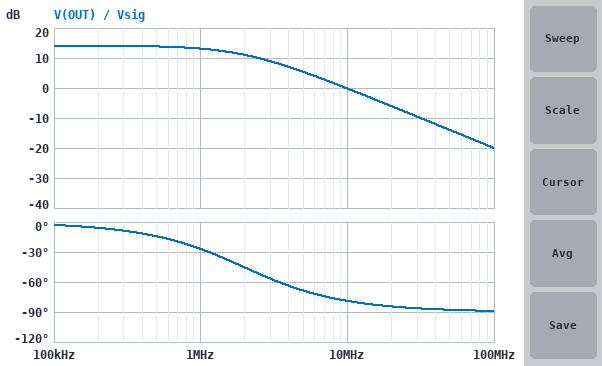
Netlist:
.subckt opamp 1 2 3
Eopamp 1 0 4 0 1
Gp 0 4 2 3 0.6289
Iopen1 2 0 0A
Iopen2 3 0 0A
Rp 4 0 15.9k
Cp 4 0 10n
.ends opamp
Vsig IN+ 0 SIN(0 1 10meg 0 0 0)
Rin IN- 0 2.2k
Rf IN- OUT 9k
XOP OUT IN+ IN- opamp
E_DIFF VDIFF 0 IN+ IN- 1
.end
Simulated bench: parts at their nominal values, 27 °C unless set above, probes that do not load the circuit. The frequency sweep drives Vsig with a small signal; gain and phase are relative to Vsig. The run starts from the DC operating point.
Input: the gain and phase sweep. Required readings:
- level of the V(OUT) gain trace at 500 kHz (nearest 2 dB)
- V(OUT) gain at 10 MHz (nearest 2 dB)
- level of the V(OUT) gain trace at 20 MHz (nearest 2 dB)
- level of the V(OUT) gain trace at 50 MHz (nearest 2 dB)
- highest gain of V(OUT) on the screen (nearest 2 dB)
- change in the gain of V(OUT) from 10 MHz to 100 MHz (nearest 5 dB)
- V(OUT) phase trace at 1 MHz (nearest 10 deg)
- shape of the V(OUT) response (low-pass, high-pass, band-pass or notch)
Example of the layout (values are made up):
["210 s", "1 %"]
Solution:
["14 dB", "0 dB", "-6 dB", "-14 dB", "14 dB", "-20 dB", "-30 deg", "low-pass"]
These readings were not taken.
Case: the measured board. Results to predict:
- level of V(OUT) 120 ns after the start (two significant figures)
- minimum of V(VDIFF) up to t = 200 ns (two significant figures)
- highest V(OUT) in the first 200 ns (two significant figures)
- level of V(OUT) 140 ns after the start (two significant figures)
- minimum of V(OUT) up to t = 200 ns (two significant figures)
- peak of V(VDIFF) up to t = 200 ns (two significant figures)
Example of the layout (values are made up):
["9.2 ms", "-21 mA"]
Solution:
["100 mV", "-1.1 V", "1.5 V", "1.1 V", "-900 mV", "940 mV"]
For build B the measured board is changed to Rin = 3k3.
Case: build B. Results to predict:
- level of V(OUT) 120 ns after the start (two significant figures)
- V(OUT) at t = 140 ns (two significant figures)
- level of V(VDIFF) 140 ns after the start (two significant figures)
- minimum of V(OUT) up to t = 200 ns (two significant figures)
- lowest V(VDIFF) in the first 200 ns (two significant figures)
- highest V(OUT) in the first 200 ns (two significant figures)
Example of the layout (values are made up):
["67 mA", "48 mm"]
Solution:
["73 mV", "990 mV", "320 mV", "-930 mV", "-1.0 V", "1.4 V"]
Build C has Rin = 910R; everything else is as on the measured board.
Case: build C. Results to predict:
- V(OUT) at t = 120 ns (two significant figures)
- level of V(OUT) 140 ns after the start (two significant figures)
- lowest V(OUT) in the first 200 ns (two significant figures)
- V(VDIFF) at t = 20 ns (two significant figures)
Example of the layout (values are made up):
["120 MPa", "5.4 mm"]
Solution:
["280 mV", "1.3 V", "-680 mV", "890 mV"]
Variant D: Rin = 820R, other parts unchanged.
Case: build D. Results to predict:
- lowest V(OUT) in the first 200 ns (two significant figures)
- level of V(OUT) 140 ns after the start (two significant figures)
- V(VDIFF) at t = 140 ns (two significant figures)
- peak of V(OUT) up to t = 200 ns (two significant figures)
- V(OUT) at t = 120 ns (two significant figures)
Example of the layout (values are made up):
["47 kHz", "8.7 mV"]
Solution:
["-650 mV", "1.3 V", "480 mV", "1.8 V", "300 mV"]
